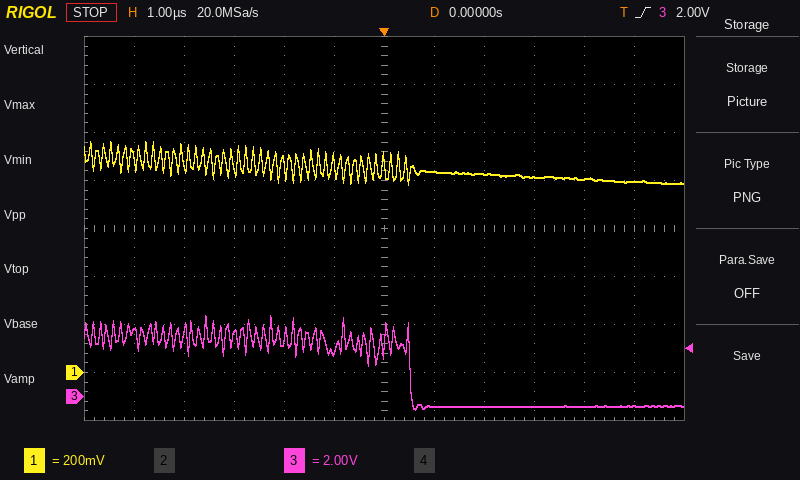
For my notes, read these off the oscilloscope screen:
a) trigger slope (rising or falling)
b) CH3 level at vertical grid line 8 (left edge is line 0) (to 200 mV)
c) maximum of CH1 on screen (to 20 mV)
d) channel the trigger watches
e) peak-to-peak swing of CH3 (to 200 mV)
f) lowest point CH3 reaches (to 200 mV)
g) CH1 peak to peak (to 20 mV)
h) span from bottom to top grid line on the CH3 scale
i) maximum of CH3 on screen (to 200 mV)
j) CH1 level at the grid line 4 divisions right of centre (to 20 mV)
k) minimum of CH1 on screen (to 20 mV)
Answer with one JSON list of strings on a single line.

["rising", "-400 mV", "960 mV", "CH3", "4.0 V", "-600 mV", "180 mV", "16 V", "3.4 V", "800 mV", "780 mV"]
